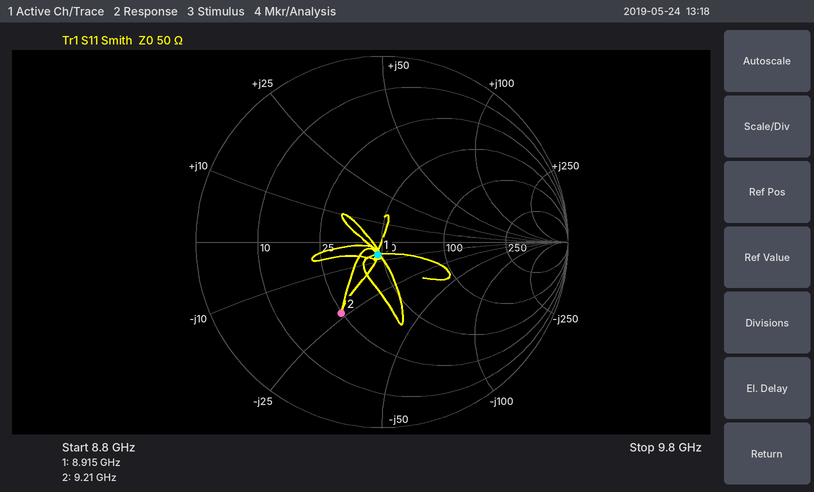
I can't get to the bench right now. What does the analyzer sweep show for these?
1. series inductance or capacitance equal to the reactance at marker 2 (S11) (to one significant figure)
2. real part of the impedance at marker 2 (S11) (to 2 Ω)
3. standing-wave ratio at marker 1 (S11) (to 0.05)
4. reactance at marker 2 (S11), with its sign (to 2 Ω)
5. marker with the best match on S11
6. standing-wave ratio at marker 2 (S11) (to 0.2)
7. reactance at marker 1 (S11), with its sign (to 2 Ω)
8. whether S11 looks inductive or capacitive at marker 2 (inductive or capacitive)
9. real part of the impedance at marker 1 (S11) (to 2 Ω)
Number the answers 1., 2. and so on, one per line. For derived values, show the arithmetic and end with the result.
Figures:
1. C = 1/(2π × 9.21 GHz × 24 Ω) ≈ 720 fF, so 700 fF to one significant figure
2. 24 Ω
3. 1.15
4. -24 Ω
5. marker 1
6. 2.6
7. -6 Ω
8. capacitive
9. 48 Ω
